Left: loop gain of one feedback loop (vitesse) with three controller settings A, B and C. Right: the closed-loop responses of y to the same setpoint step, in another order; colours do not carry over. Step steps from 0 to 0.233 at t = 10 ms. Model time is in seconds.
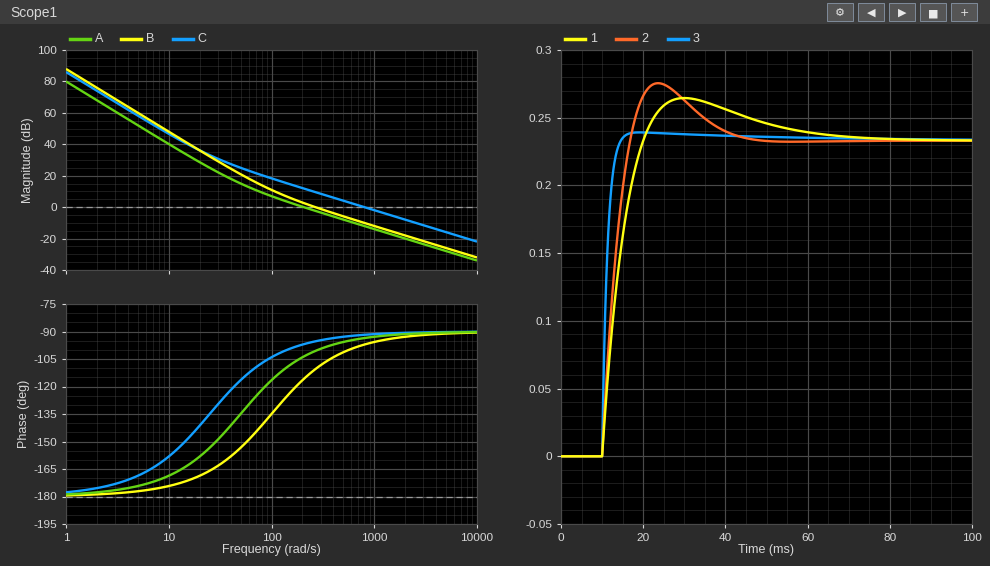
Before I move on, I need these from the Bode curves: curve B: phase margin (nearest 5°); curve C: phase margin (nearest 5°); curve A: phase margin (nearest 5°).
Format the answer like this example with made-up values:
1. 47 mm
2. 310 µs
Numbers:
1. 70°
2. 90°
3. 75°
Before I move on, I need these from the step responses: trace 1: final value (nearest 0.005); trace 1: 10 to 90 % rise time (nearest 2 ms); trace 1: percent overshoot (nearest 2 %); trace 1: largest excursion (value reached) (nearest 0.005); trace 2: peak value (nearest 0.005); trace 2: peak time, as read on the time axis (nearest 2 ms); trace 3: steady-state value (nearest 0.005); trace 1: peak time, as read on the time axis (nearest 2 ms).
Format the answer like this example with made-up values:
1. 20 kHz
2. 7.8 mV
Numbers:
1. 0.235
2. 8 ms
3. 14 %
4. 0.265
5. 0.275
6. 24 ms
7. 0.235
8. 30 ms
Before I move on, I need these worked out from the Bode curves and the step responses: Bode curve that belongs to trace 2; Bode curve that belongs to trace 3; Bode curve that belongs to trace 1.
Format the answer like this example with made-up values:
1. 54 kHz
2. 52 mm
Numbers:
1. B
2. C
3. A
